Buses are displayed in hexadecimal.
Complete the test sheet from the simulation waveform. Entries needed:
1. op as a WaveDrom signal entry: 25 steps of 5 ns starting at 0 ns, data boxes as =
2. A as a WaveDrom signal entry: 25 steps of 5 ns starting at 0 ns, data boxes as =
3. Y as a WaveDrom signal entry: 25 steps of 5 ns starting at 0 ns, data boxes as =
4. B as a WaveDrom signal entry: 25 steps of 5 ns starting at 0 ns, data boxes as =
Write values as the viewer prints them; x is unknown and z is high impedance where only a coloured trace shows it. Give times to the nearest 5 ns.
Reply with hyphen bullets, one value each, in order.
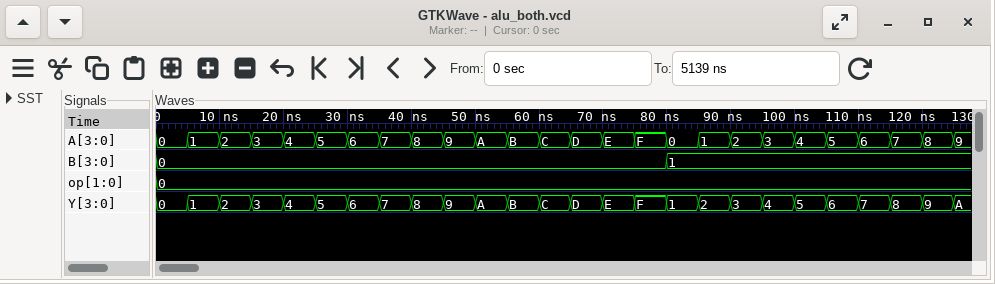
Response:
- {name: 'op', wave: '=........................', data: '0'}
- {name: 'A', wave: '=========================', data: '0 1 2 3 4 5 6 7 8 9 A B C D E F 0 1 2 3 4 5 6 7 8'}
- {name: 'Y', wave: '=========================', data: '0 1 2 3 4 5 6 7 8 9 A B C D E F 1 2 3 4 5 6 7 8 9'}
- {name: 'B', wave: '=...............=........', data: '0 1'}
